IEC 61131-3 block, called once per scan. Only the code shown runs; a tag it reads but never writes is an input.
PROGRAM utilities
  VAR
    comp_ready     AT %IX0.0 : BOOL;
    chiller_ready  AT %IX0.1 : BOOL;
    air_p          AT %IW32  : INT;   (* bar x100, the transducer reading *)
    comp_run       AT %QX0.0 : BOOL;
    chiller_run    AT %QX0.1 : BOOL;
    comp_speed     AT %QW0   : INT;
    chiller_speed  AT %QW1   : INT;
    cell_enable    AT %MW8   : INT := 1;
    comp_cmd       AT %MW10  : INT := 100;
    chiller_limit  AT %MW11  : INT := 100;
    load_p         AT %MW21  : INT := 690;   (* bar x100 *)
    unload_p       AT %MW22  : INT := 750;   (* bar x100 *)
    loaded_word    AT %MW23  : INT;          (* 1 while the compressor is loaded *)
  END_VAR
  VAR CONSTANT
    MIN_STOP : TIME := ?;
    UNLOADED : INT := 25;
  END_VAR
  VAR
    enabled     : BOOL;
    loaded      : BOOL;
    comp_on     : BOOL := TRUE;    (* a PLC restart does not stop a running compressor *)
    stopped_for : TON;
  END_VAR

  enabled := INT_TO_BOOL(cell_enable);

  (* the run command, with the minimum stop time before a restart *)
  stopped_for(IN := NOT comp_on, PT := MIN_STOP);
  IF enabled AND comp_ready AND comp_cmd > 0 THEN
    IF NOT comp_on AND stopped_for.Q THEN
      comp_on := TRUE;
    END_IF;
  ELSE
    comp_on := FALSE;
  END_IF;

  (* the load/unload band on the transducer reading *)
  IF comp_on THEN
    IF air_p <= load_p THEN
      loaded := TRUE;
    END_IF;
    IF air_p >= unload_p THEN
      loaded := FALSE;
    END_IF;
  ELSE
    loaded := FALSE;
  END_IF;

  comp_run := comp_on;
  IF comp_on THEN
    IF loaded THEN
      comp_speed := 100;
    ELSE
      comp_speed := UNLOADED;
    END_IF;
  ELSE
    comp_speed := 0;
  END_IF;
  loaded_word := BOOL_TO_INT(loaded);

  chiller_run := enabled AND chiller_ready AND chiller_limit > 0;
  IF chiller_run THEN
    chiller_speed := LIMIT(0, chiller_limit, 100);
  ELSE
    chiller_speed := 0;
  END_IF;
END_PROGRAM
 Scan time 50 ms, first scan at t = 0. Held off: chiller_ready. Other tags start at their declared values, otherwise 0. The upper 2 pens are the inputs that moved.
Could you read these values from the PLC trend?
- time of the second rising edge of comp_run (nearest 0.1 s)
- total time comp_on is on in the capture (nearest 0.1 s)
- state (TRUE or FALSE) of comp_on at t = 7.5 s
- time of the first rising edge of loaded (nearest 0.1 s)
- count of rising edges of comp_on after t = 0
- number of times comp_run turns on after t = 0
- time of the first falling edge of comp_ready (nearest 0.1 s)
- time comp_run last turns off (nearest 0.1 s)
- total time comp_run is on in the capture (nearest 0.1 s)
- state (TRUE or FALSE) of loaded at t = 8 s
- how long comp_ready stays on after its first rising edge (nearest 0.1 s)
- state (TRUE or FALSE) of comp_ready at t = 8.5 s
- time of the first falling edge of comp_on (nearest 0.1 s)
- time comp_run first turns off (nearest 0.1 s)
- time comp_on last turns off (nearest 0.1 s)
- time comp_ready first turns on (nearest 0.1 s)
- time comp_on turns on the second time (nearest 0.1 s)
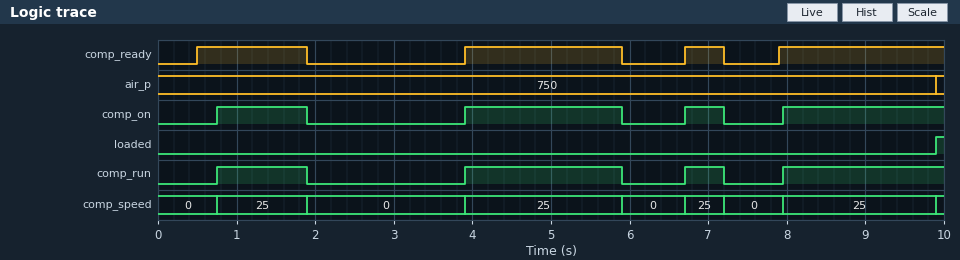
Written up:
3.9 s
5.7 s
FALSE
9.9 s
4
4
1.9 s
7.2 s
5.7 s
FALSE
1.4 s
TRUE
1.9 s
1.9 s
7.2 s
0.5 s
3.9 s
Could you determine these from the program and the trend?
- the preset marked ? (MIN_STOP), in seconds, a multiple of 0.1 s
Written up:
0.7 s
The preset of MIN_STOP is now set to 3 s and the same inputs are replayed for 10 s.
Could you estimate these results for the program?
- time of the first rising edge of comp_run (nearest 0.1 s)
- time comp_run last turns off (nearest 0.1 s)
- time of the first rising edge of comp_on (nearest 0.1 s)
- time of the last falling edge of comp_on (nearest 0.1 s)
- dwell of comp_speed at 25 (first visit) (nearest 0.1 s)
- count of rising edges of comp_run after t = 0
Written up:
3.9 s
5.9 s
3.9 s
5.9 s
2.0 s
2
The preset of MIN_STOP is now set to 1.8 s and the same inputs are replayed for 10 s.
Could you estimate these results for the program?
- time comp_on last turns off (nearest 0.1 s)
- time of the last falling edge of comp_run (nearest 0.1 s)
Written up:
5.9 s
5.9 s
